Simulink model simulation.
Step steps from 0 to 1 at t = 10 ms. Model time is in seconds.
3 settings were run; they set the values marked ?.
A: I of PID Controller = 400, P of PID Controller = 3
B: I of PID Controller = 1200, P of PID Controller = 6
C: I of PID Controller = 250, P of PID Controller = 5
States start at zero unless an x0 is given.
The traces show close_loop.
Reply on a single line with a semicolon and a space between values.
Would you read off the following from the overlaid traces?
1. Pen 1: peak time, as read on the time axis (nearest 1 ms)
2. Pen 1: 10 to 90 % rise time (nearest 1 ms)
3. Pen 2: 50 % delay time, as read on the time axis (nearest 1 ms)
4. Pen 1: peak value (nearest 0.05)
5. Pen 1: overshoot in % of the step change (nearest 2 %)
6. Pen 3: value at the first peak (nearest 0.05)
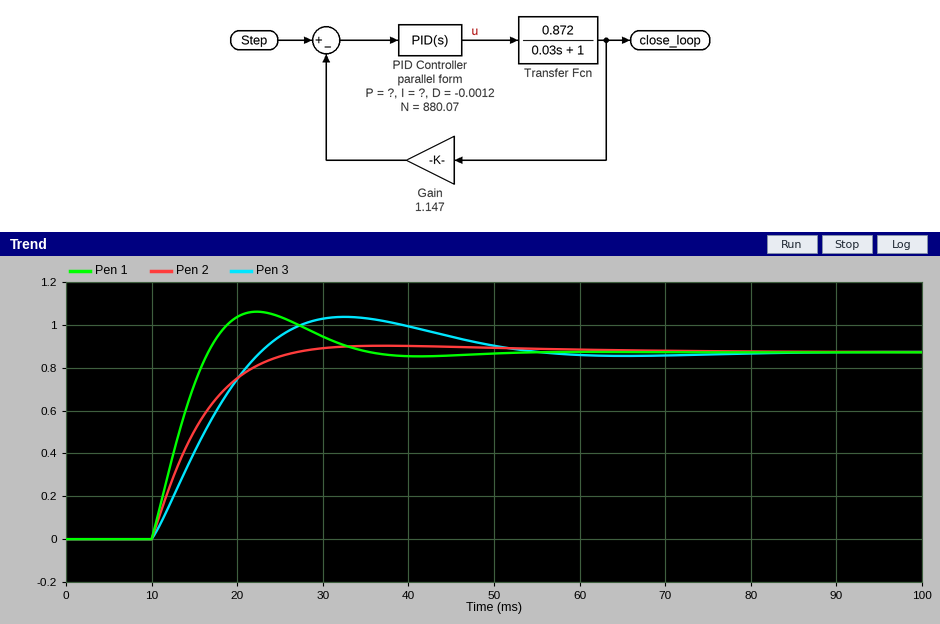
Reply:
22 ms; 5 ms; 14 ms; 1.05; 22 %; 1.05
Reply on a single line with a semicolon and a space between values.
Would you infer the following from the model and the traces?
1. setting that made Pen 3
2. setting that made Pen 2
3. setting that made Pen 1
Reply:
A; C; B
